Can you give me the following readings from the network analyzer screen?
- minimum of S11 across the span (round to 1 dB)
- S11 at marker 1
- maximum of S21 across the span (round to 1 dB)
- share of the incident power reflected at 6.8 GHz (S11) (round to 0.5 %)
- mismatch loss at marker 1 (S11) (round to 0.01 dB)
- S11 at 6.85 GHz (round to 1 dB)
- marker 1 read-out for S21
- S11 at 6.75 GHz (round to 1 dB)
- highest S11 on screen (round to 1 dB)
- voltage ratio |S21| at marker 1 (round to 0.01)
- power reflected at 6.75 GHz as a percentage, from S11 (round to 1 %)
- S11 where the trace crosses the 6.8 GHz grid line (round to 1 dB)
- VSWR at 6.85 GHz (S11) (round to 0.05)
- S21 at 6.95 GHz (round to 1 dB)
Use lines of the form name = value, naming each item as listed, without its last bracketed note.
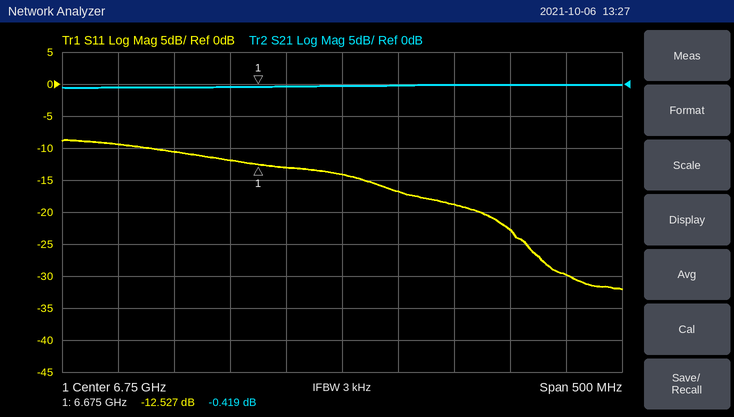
minimum of S11 across the span = -32 dB
S11 at marker 1 = -12.527 dB
maximum of S21 across the span = 0 dB
share of the incident power reflected at 6.8 GHz (S11) = 2.0 %
mismatch loss at marker 1 (S11) = 0.25 dB
S11 at 6.85 GHz = -19 dB
marker 1 read-out for S21 = -0.419 dB
S11 at 6.75 GHz = -14 dB
highest S11 on screen = -9 dB
voltage ratio |S21| at marker 1 = 0.95
power reflected at 6.75 GHz as a percentage, from S11 = 4 %
S11 where the trace crosses the 6.8 GHz grid line = -17 dB
VSWR at 6.85 GHz (S11) = 1.25
S21 at 6.95 GHz = 0 dB
